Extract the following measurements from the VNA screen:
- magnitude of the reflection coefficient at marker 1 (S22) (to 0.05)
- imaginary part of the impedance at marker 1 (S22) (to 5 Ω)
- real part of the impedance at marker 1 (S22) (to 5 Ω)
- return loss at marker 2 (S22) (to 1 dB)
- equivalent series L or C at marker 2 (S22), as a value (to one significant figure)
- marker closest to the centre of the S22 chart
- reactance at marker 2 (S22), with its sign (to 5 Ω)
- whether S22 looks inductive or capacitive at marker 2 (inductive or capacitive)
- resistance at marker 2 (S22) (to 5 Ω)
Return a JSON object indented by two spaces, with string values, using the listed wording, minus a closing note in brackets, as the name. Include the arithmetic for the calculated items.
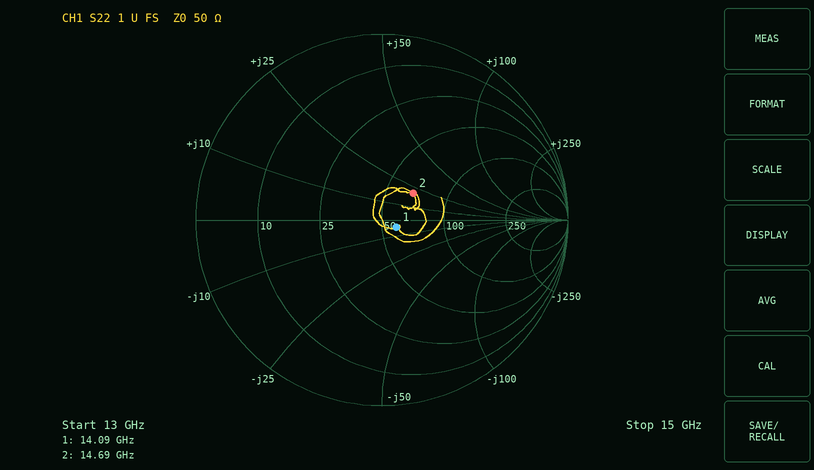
{
  "magnitude of the reflection coefficient at marker 1 (S22)": "0.10",
  "imaginary part of the impedance at marker 1 (S22)": "-5 Ω",
  "real part of the impedance at marker 1 (S22)": "60 Ω",
  "return loss at marker 2 (S22)": "13 dB",
  "equivalent series L or C at marker 2 (S22), as a value": "L = 20 Ω/(2π × 14.69 GHz) ≈ 217 pH, so 200 pH to one significant figure",
  "marker closest to the centre of the S22 chart": "marker 1",
  "reactance at marker 2 (S22), with its sign": "+20 Ω",
  "whether S22 looks inductive or capacitive at marker 2": "inductive",
  "resistance at marker 2 (S22)": "65 Ω"
}
